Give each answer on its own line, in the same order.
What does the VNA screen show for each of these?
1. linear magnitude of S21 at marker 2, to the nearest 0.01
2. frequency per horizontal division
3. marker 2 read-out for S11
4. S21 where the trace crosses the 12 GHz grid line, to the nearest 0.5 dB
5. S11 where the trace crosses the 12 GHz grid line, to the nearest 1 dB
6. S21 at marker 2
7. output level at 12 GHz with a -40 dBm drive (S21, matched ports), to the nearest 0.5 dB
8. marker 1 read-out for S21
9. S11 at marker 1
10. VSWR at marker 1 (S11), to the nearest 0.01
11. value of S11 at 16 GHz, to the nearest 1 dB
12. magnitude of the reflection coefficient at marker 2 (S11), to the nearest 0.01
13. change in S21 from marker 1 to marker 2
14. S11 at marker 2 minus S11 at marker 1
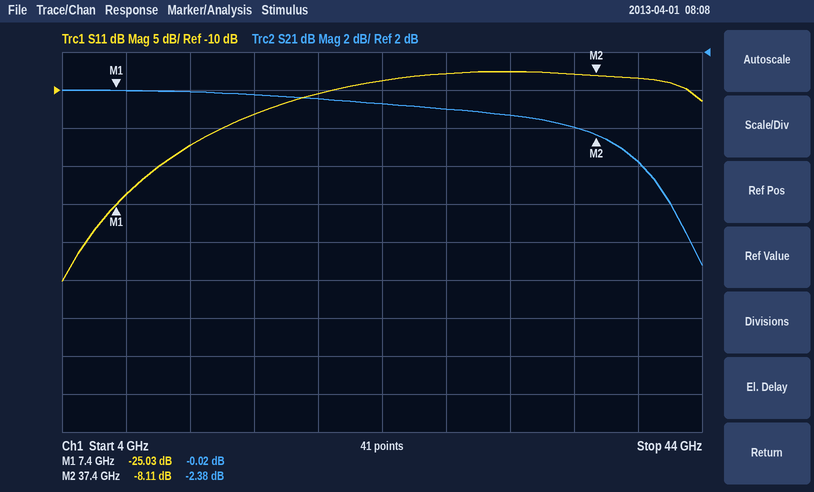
0.76
4 GHz
-8.11 dB
0.0 dB
-17 dB
-2.38 dB
-40.0 dBm
-0.02 dB
-25.03 dB
1.12
-13 dB
0.39
-2.36 dB
16.92 dB
